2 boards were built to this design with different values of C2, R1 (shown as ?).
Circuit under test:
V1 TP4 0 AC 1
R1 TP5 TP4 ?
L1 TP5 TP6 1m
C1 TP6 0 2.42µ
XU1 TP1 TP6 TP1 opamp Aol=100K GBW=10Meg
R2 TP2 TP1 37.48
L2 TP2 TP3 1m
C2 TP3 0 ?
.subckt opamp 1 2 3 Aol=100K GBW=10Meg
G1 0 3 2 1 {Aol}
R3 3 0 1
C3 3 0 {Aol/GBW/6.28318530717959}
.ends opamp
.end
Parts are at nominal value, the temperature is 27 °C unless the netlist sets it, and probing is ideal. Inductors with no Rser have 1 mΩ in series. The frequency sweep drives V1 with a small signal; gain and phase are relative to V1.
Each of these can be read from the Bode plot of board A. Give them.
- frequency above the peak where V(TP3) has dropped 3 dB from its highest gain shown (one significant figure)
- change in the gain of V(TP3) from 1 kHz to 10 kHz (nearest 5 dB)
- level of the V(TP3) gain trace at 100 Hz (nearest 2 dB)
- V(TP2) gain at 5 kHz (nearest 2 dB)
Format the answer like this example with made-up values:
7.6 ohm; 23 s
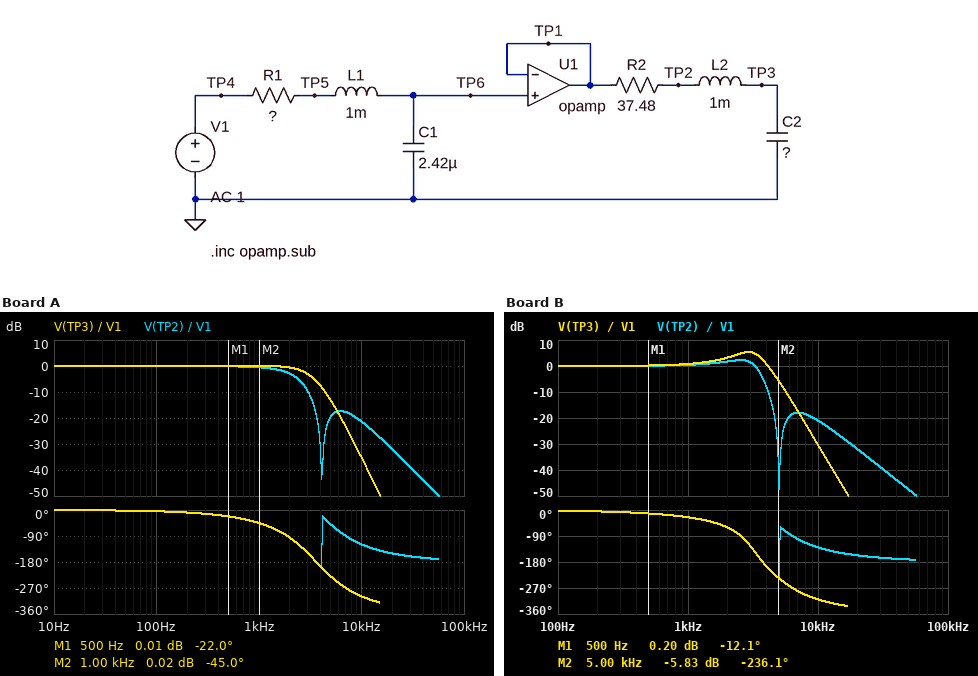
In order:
3 kHz; -35 dB; 0 dB; -20 dB
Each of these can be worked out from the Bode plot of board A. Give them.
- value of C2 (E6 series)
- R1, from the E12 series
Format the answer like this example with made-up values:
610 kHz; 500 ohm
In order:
1.5 µF; 27 Ω
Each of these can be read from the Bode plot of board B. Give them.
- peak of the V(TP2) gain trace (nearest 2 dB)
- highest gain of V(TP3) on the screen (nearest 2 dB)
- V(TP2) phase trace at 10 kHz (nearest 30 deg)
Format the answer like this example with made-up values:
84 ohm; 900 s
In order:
2 dB; 6 dB; -120 deg
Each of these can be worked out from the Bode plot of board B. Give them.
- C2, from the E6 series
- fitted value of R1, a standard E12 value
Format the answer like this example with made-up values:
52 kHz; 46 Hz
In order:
1 µF; 12 Ω
